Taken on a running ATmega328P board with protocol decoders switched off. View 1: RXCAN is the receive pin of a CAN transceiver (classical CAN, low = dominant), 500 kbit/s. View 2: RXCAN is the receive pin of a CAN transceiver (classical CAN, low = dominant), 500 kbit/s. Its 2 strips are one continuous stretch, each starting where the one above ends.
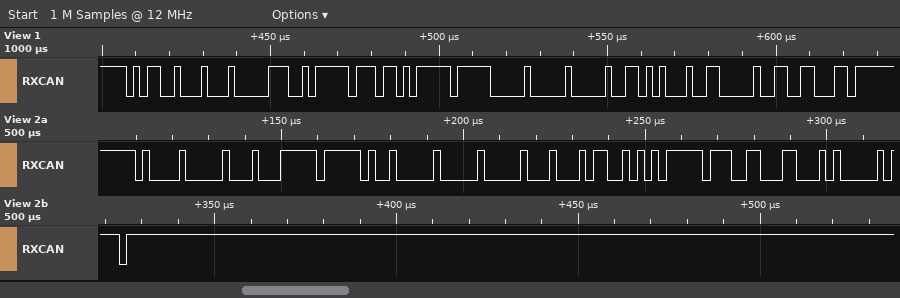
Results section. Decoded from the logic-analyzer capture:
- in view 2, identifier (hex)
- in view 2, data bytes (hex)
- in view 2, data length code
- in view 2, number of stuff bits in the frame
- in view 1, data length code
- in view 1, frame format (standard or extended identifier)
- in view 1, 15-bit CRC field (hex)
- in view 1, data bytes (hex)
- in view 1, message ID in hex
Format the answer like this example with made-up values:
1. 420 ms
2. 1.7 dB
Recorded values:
1. 0x420
2. FF E4 00 00 8B 2A FF 31
3. 8
4. 8
5. 8
6. standard
7. 0x0331
8. 32 FF 6B FF 00 00 D4 4C
9. 0x591
